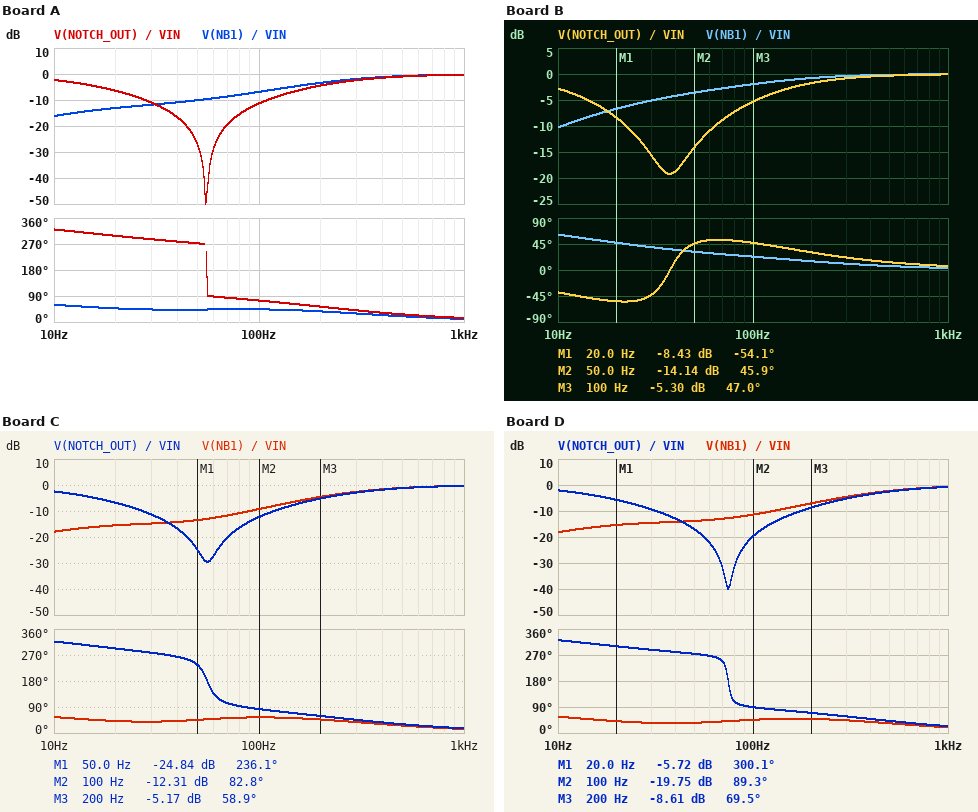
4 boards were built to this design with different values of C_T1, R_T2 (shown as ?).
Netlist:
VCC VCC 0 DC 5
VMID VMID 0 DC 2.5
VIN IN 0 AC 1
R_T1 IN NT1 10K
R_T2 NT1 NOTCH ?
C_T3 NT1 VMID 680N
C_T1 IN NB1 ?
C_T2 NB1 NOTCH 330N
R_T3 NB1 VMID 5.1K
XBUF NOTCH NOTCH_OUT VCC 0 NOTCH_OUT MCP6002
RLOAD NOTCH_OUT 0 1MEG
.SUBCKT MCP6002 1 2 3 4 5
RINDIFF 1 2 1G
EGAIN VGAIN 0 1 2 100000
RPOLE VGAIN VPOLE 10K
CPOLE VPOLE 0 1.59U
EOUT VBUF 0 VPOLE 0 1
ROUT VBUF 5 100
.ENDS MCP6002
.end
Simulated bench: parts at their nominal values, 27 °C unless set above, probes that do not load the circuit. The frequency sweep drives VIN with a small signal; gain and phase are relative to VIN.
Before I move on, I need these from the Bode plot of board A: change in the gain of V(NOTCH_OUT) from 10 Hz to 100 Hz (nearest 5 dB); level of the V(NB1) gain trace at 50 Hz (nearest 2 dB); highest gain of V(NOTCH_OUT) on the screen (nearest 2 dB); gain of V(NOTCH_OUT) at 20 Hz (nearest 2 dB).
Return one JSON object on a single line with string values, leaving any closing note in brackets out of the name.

{"change in the gain of V(NOTCH_OUT) from 10 Hz to 100 Hz": "-10 dB", "level of the V(NB1) gain trace at 50 Hz": "-10 dB", "highest gain of V(NOTCH_OUT) on the screen": "0 dB", "gain of V(NOTCH_OUT) at 20 Hz": "-6 dB"}
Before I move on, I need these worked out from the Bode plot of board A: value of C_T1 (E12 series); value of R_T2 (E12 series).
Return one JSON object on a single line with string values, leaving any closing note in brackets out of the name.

{"value of C_T1": "270 nF", "value of R_T2": "8.2 kΩ"}
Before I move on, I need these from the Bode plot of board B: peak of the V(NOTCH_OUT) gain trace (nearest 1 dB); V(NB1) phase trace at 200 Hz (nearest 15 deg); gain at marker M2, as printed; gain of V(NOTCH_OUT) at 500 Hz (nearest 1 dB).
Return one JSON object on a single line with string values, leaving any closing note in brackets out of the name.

{"peak of the V(NOTCH_OUT) gain trace": "0 dB", "V(NB1) phase trace at 200 Hz": "15 deg", "gain at marker M2, as printed": "-14.14 dB", "gain of V(NOTCH_OUT) at 500 Hz": "0 dB"}
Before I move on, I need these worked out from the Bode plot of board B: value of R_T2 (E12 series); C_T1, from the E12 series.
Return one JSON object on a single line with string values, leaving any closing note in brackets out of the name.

{"value of R_T2": "8.2 kΩ", "C_T1, from the E12 series": "820 nF"}
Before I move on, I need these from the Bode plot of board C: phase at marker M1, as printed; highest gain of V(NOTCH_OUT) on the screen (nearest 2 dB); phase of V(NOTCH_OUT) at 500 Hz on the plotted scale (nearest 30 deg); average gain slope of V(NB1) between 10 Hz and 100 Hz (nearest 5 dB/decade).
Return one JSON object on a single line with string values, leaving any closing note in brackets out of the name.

{"phase at marker M1, as printed": "236.1 deg", "highest gain of V(NOTCH_OUT) on the screen": "0 dB", "phase of V(NOTCH_OUT) at 500 Hz on the plotted scale": "30 deg", "average gain slope of V(NB1) between 10 Hz and 100 Hz": "10 dB/decade"}
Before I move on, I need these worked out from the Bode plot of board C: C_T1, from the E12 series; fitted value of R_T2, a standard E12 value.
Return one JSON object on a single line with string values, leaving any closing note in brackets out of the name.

{"C_T1, from the E12 series": "180 nF", "fitted value of R_T2, a standard E12 value": "12 kΩ"}
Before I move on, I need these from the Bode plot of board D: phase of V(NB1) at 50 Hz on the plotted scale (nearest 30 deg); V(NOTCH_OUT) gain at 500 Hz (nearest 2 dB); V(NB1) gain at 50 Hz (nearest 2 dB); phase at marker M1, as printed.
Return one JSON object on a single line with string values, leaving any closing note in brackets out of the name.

{"phase of V(NB1) at 50 Hz on the plotted scale": "30 deg", "V(NOTCH_OUT) gain at 500 Hz": "-2 dB", "V(NB1) gain at 50 Hz": "-14 dB", "phase at marker M1, as printed": "300.1 deg"}
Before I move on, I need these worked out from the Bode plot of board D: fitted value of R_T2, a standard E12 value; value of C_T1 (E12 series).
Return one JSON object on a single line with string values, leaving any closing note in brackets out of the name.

{"fitted value of R_T2, a standard E12 value": "6.8 kΩ", "value of C_T1": "150 nF"}
